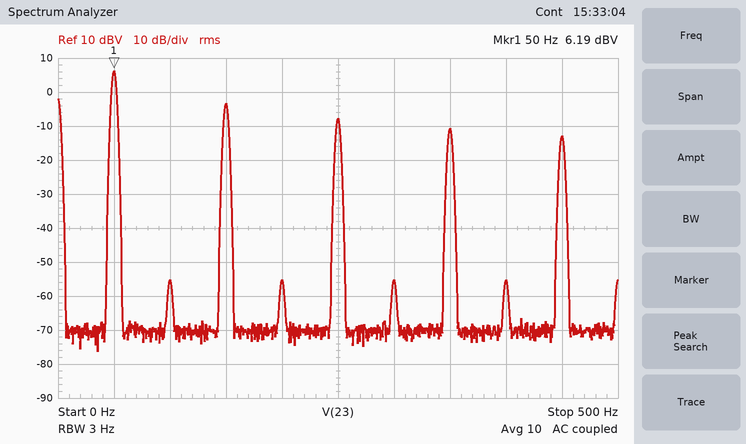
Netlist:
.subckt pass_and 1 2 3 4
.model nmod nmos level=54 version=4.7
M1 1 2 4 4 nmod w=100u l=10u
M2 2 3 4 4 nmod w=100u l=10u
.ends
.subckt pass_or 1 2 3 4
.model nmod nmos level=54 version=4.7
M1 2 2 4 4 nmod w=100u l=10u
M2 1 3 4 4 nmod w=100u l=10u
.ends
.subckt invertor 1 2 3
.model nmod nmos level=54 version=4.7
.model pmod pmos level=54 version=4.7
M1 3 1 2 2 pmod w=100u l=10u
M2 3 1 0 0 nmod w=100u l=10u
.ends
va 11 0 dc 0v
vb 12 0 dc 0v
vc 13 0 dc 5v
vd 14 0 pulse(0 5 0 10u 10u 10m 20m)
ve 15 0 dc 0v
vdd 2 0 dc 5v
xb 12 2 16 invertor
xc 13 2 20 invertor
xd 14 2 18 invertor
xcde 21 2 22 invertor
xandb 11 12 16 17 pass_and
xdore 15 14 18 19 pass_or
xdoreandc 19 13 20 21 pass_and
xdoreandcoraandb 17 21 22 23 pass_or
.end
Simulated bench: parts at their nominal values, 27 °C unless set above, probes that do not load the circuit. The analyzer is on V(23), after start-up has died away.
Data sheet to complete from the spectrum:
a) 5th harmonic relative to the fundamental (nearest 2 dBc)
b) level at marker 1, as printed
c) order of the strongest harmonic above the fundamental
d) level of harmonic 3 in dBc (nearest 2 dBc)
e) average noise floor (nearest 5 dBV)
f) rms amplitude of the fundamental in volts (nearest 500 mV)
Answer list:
-14 dBc
6.19 dBV
3
-10 dBc
-70 dBV
2.0 V
